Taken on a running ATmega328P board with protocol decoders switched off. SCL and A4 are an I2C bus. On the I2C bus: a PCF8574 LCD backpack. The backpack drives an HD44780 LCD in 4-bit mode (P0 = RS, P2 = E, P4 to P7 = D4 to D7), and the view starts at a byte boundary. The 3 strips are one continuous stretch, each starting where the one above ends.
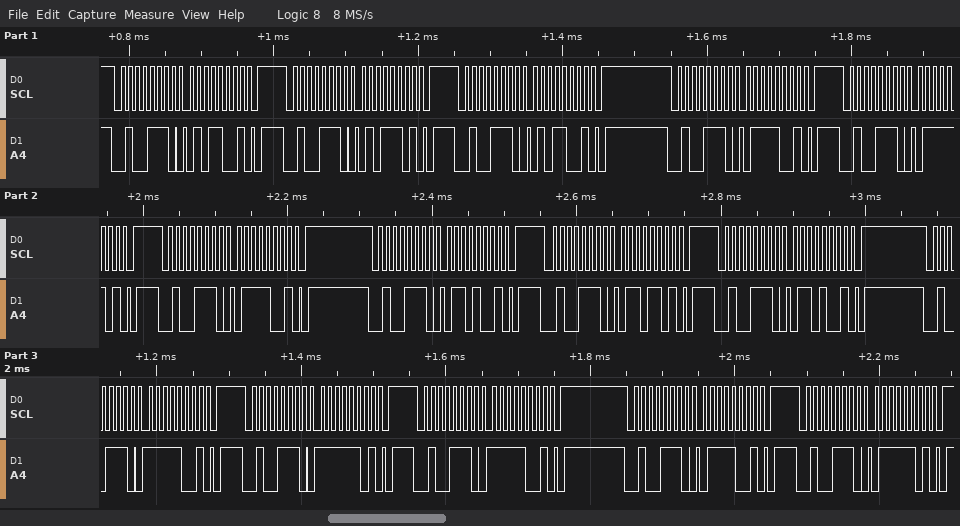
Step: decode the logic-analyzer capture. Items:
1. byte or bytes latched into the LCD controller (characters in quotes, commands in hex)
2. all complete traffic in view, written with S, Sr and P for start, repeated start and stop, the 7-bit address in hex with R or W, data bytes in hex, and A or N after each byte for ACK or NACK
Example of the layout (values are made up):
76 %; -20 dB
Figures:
'W' 'o'; S 27W A 59 A P S 27W A 5D A P S 27W A 59 A P S 27W A 79 A P S 27W A 7D A P S 27W A 79 A P S 27W A 69 A P S 27W A 6D A P S 27W A 69 A P S 27W A F9 A P S 27W A FD A P S 27W A F9 A P S 27W A 79 A P S 27W A 7D A P
